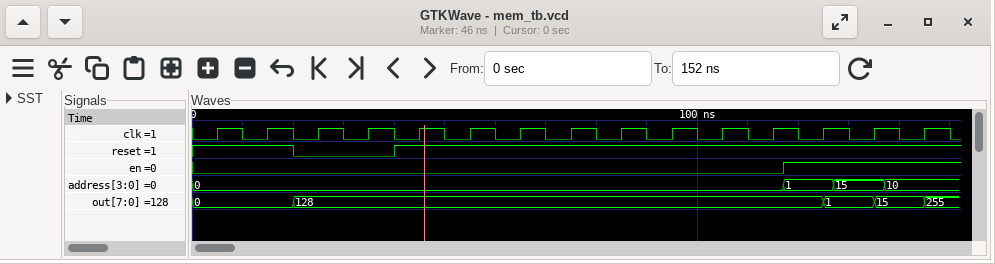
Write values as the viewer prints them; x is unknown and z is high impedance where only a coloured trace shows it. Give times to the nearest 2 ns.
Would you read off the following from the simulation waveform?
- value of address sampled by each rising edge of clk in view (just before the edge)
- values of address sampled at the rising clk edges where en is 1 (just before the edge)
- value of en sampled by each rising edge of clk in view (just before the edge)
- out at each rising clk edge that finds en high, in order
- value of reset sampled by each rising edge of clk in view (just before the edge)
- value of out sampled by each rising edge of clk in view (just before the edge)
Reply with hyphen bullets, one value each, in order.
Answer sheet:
- 0, 0, 0, 0, 0, 0, 0, 0, 0, 0, 0, 0, 1, 15, 10
- 1, 15, 10
- 0 0 0 0 0 0 0 0 0 0 0 0 1 1 1
- 128, 1, 15
- 1 1 0 0 1 1 1 1 1 1 1 1 1 1 1
- 0, 0, 128, 128, 128, 128, 128, 128, 128, 128, 128, 128, 128, 1, 15
